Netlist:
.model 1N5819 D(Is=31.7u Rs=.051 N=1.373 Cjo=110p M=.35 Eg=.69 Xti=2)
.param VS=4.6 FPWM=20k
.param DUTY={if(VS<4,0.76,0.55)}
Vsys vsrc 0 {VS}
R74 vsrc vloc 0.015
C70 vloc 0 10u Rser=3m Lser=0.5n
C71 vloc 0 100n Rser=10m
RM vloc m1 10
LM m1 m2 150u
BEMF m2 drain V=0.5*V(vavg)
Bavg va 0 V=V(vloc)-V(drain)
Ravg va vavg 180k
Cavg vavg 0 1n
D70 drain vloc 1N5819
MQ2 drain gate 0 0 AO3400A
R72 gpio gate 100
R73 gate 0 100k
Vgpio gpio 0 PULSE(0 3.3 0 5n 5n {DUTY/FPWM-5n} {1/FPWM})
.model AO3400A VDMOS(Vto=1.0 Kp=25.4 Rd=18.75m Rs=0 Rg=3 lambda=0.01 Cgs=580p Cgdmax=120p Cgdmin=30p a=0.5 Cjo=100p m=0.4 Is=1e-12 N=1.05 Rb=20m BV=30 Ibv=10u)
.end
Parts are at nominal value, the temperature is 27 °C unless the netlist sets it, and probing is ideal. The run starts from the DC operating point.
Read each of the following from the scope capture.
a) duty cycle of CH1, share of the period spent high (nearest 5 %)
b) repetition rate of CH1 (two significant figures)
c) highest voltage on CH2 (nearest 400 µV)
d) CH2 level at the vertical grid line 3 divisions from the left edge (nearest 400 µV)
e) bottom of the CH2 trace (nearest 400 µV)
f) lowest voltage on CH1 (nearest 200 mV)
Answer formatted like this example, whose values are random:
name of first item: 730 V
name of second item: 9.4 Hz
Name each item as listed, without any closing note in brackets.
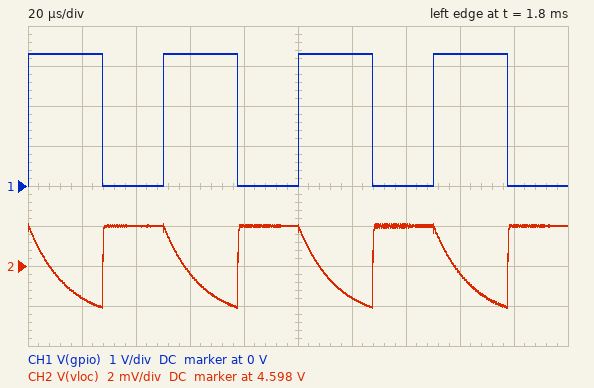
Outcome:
duty cycle of CH1, share of the period spent high: 55 %
repetition rate of CH1: 20 kHz
highest voltage on CH2: 4.6000 V
CH2 level at the vertical grid line 3 divisions from the left edge: 4.5976 V
bottom of the CH2 trace: 4.5960 V
lowest voltage on CH1: 0 V
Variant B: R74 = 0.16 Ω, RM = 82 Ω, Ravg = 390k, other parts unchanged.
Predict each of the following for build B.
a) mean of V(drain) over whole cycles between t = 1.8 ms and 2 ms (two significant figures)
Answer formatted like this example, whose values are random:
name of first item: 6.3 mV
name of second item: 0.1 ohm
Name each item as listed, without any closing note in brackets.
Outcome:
mean of V(drain) over whole cycles between t = 1.8 ms and 2 ms: 1.4 V
